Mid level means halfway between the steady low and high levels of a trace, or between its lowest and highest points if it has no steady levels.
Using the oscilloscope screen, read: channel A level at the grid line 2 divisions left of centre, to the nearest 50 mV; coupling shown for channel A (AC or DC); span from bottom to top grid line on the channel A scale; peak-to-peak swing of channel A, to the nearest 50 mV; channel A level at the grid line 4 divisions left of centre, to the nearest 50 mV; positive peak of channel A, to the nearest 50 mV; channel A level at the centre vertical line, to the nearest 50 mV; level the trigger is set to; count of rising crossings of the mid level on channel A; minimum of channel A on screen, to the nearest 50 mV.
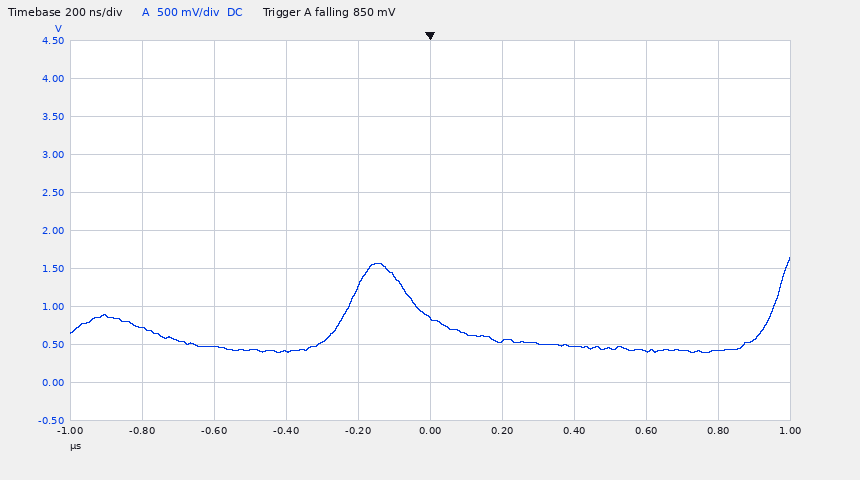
400 mV
DC
5 V
1.25 V
700 mV
1.65 V
850 mV
850 mV
2
400 mV
